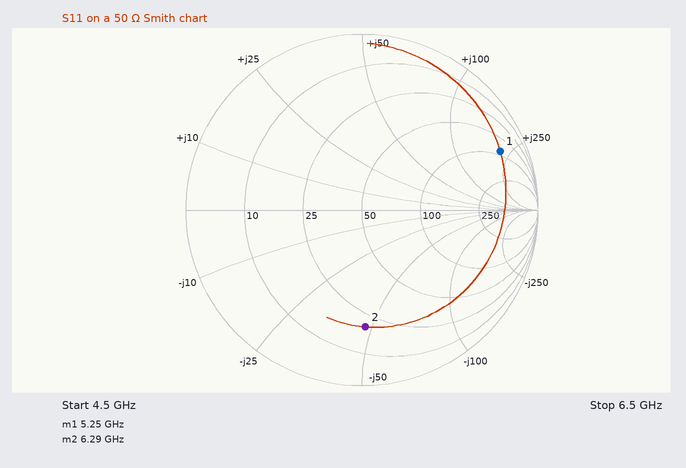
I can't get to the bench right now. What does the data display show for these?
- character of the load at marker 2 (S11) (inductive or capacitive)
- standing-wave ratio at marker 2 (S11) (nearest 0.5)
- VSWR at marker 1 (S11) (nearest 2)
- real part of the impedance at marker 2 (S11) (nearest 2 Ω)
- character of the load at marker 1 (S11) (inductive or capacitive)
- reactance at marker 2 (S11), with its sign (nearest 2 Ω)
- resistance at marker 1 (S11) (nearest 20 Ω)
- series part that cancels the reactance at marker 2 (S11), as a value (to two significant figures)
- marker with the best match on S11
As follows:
capacitive
5.0
12
20 Ω
inductive
-48 Ω
80 Ω
1.2 nH
marker 2
